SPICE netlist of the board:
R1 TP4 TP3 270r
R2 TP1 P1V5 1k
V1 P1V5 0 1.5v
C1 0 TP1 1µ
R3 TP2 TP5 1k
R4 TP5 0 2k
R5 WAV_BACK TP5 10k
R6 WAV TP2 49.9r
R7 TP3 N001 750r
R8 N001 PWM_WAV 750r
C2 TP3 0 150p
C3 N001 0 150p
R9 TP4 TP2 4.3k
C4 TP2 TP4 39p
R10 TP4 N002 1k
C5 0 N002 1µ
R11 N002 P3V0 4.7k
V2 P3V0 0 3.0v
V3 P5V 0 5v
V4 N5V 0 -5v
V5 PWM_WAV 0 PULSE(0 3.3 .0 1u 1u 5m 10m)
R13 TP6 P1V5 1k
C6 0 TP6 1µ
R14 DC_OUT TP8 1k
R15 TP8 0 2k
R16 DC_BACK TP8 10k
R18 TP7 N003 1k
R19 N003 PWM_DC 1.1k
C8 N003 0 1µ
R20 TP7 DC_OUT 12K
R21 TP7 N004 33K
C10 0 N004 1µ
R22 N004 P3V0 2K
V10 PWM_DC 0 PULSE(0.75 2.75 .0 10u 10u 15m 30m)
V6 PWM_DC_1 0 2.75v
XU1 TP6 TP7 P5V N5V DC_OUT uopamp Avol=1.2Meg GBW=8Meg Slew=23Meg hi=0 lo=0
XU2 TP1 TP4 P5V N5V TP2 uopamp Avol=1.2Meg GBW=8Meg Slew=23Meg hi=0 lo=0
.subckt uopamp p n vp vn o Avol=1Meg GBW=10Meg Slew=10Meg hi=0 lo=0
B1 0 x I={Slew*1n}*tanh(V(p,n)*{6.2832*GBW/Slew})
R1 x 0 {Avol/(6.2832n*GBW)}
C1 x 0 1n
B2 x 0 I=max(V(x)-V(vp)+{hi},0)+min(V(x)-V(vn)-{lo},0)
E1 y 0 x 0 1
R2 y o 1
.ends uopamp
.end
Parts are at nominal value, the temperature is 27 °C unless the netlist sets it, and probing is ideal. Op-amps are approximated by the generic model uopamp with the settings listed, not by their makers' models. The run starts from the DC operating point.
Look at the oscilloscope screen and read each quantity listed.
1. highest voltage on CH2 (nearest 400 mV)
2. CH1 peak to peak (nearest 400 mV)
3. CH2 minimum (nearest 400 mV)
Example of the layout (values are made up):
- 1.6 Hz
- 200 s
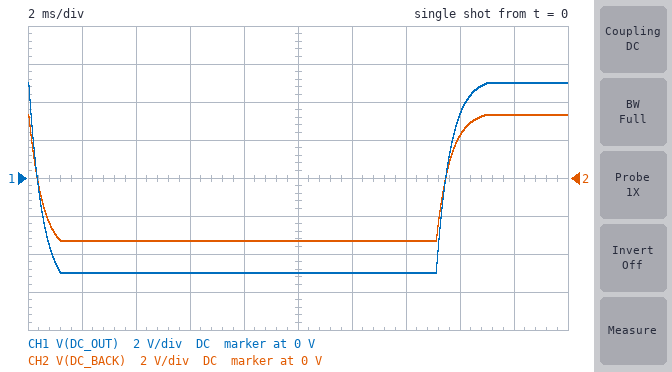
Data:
- 3.2 V
- 10.0 V
- -3.2 V
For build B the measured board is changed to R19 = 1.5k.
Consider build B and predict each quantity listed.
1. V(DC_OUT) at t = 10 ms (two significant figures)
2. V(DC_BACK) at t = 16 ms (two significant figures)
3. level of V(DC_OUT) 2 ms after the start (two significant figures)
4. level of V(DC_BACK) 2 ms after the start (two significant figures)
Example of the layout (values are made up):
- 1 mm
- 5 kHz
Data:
- -5.0 V
- 1.8 V
- -4.7 V
- -3.1 V
